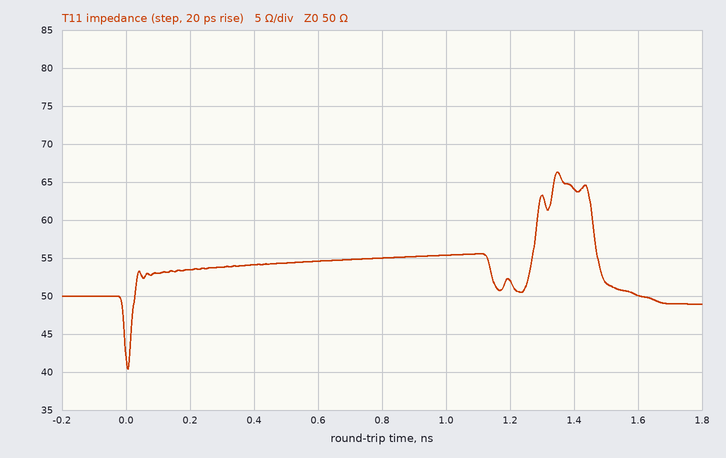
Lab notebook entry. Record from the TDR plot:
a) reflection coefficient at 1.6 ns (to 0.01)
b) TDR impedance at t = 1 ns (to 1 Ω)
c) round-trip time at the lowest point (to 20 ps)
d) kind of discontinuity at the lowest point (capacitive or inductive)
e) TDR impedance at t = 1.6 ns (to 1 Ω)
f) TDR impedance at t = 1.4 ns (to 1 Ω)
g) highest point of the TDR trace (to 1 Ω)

0.00
55 Ω
0 ps
capacitive
50 Ω
64 Ω
66 Ω
